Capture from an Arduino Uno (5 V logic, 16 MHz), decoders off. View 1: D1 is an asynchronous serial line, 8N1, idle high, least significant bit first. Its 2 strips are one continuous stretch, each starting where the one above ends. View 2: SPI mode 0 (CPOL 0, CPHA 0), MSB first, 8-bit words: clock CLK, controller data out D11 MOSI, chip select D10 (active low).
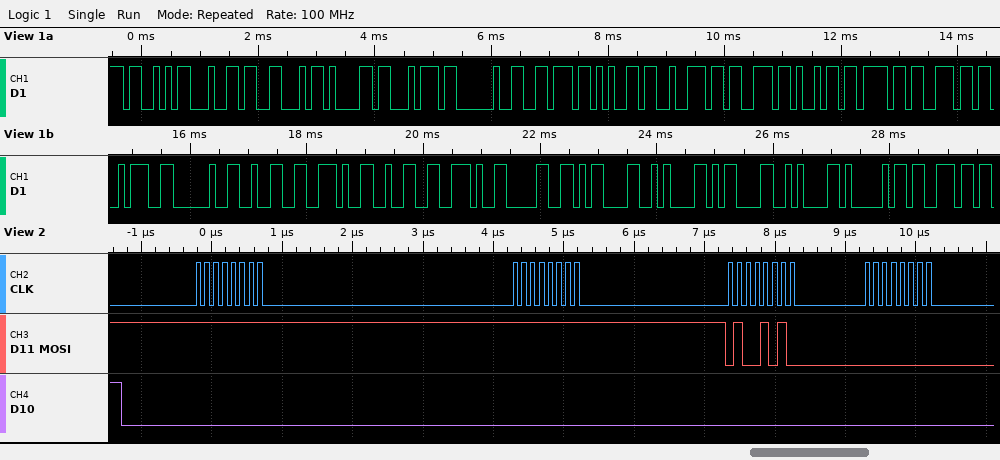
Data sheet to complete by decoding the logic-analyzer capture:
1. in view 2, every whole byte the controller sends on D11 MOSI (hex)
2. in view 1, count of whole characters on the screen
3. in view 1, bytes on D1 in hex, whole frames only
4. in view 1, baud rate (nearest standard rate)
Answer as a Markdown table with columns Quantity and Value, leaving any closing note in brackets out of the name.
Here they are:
| Quantity | Value |
|---|---|
| in view 2, every whole byte the controller sends on D11 MOSI | FF FF 4A 00 |
| in view 1, count of whole characters on the screen | 26 |
| in view 1, bytes on D1 in hex, whole frames only | 53 64 46 61 74 20 76 65 72 73 69 6F 6E 3A 20 32 2E 32 2E 30 0D 0A 0D 0A 41 73 |
| in view 1, baud rate | 9600 baud |
